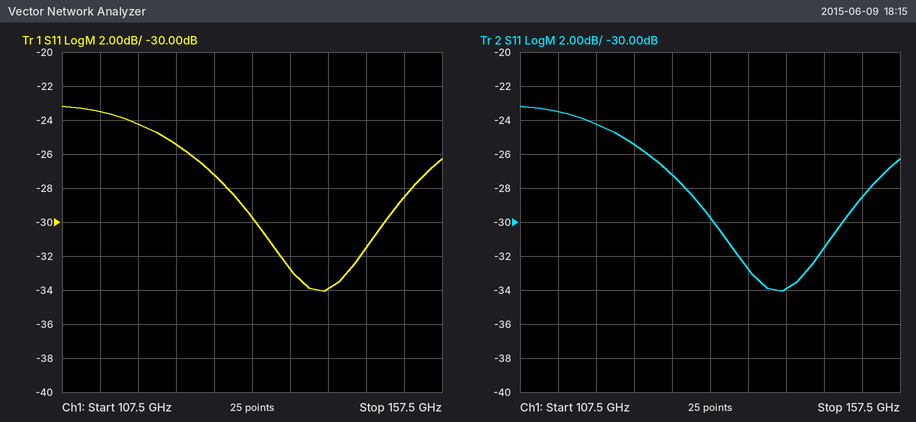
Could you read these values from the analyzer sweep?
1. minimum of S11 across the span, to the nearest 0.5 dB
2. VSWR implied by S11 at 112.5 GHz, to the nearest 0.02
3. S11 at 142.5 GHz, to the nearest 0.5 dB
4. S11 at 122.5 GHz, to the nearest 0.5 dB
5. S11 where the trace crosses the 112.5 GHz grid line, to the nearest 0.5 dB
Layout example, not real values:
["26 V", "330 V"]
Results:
["-34.0 dB", "1.14", "-34.0 dB", "-25.5 dB", "-23.5 dB"]
